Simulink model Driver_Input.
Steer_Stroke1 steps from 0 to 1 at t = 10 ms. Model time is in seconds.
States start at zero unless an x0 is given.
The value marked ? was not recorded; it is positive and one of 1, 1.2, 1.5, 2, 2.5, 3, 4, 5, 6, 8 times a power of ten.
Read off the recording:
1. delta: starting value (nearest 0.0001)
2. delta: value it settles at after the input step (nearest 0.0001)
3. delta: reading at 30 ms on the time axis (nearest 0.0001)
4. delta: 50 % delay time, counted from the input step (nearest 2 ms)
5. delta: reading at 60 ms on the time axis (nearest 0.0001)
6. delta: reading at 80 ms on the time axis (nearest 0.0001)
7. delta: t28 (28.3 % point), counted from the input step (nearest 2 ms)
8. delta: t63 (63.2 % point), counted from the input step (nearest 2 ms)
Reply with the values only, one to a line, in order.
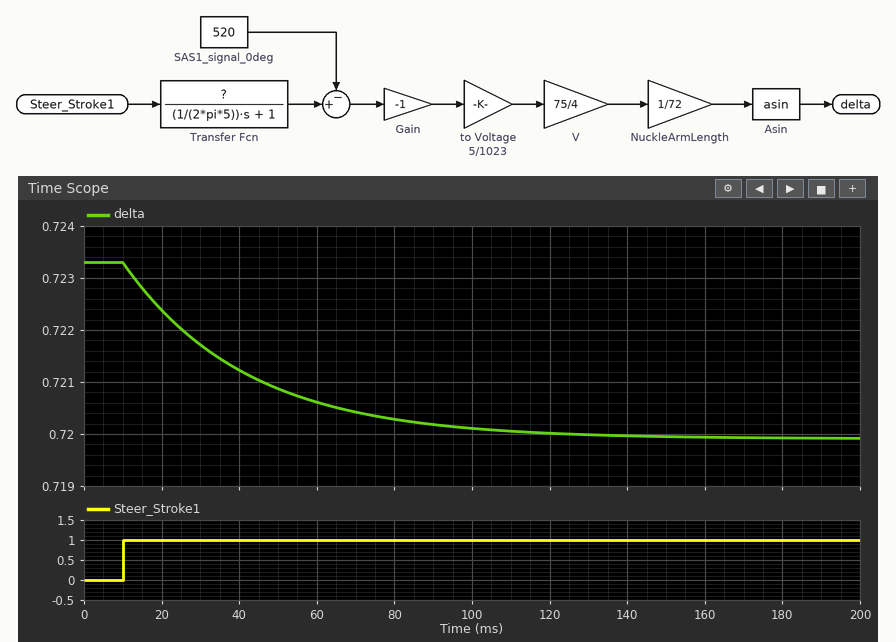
0.7233
0.7199
0.7217
22 ms
0.7206
0.7203
10 ms
32 ms
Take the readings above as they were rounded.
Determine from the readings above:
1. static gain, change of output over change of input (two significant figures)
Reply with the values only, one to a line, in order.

-0.0034
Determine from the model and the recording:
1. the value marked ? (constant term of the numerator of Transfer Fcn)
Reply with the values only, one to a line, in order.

2
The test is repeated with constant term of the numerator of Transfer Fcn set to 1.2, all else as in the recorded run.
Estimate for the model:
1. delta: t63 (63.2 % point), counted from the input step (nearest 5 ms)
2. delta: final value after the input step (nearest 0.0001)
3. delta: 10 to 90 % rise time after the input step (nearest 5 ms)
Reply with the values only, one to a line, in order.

30 ms
0.7213
70 ms
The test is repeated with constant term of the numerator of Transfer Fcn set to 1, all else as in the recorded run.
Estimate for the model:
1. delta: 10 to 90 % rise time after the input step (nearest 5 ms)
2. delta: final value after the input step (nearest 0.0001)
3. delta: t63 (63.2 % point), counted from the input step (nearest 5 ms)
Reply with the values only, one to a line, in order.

70 ms
0.7216
30 ms
